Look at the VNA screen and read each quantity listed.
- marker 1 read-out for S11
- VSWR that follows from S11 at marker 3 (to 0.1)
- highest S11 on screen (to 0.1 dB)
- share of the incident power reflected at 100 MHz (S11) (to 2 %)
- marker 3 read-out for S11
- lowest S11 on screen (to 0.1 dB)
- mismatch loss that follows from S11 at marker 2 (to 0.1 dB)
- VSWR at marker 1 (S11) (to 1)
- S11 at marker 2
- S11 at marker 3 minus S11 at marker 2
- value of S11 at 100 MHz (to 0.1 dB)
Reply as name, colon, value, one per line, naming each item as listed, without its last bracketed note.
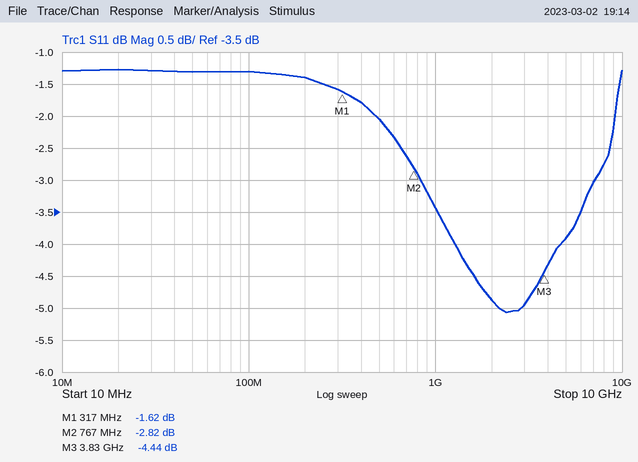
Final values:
marker 1 read-out for S11: -1.62 dB
VSWR that follows from S11 at marker 3: 4.0
highest S11 on screen: -1.3 dB
share of the incident power reflected at 100 MHz (S11): 74 %
marker 3 read-out for S11: -4.44 dB
lowest S11 on screen: -5.1 dB
mismatch loss that follows from S11 at marker 2: 3.2 dB
VSWR at marker 1 (S11): 11
S11 at marker 2: -2.82 dB
S11 at marker 3 minus S11 at marker 2: -1.62 dB
value of S11 at 100 MHz: -1.3 dB
